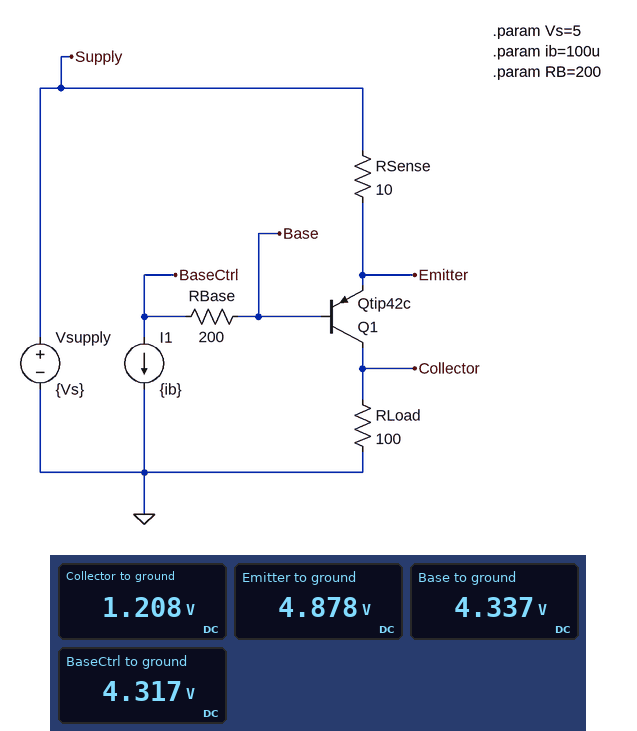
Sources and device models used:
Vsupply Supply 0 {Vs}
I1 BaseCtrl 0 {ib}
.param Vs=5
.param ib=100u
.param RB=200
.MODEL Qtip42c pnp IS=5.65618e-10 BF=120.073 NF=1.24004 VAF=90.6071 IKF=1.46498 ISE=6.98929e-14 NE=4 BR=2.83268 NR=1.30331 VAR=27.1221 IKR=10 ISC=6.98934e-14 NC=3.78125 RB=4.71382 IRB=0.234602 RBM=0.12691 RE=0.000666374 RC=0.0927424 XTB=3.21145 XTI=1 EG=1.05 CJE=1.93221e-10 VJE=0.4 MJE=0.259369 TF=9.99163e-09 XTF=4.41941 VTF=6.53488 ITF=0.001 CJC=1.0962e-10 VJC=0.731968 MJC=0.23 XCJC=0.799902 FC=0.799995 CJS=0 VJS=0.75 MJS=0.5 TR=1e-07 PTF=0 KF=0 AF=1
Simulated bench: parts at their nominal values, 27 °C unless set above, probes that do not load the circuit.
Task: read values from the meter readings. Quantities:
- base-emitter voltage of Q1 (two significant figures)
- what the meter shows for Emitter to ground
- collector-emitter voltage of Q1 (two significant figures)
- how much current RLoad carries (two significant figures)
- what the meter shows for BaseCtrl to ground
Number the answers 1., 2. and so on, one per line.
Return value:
1. -540 mV
2. 4.878 V
3. -3.7 V
4. 12 mA
5. 4.317 V
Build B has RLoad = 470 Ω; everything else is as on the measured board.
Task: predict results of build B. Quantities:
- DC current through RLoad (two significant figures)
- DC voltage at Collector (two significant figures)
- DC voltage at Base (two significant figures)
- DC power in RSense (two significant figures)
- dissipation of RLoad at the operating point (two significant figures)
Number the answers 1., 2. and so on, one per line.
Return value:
1. 10 mA
2. 4.7 V
3. 4.4 V
4. 1.0 mW
5. 48 mW
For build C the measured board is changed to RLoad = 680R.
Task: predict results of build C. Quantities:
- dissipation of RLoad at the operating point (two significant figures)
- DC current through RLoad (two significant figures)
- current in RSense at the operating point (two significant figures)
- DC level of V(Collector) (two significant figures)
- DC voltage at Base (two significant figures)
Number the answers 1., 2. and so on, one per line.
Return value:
1. 34 mW
2. 7.1 mA
3. 7.2 mA
4. 4.8 V
5. 4.4 V
